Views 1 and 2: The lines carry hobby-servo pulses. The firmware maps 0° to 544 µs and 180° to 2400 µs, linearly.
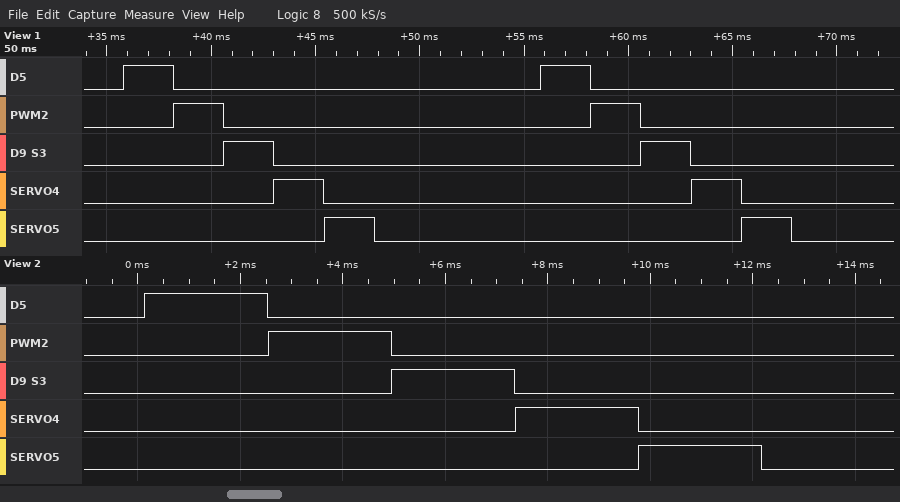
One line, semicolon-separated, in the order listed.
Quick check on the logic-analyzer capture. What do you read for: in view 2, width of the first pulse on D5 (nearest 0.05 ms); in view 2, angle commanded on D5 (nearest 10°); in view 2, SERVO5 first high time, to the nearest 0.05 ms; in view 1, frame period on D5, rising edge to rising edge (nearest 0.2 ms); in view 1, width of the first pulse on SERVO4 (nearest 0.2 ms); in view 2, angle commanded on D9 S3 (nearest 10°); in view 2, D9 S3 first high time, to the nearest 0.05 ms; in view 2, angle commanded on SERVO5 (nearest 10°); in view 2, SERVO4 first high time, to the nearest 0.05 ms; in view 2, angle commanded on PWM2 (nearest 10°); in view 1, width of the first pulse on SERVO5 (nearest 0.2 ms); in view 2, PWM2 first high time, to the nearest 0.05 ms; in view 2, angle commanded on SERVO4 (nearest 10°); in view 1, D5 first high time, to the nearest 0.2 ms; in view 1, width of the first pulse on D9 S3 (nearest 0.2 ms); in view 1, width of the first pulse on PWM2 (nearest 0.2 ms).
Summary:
2.40 ms; 180°; 2.40 ms; 20.0 ms; 2.4 ms; 180°; 2.40 ms; 180°; 2.40 ms; 180°; 2.4 ms; 2.40 ms; 180°; 2.4 ms; 2.4 ms; 2.4 ms
